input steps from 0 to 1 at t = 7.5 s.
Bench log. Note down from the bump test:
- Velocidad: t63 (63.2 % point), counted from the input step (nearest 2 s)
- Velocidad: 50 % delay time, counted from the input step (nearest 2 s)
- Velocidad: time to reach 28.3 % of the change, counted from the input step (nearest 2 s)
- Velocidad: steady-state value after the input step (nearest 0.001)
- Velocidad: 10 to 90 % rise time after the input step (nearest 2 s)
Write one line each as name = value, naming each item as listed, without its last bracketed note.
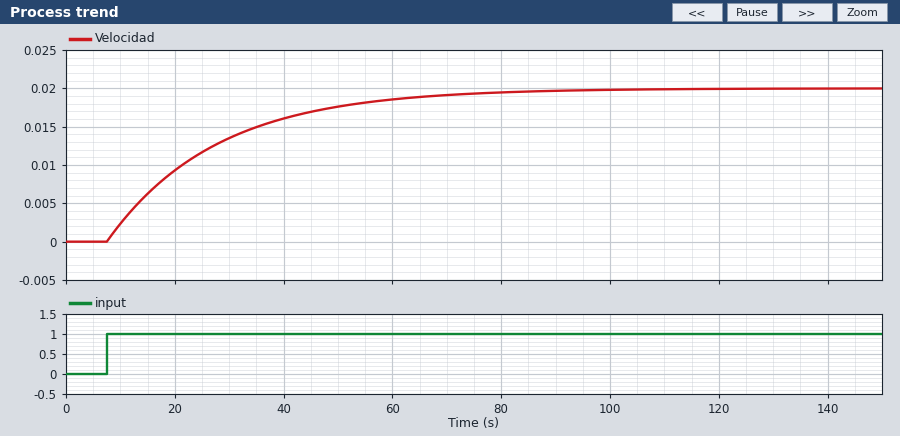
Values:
Velocidad: t63 (63.2 % point), counted from the input step = 20 s
Velocidad: 50 % delay time, counted from the input step = 14 s
Velocidad: time to reach 28.3 % of the change, counted from the input step = 6 s
Velocidad: steady-state value after the input step = 0.020
Velocidad: 10 to 90 % rise time after the input step = 44 s
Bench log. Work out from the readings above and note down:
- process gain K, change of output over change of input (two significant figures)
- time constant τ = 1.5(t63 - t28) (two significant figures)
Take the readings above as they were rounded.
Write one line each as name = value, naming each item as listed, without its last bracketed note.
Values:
process gain K, change of output over change of input = 0.020
time constant τ = 1.5(t63 - t28) = 21 s
